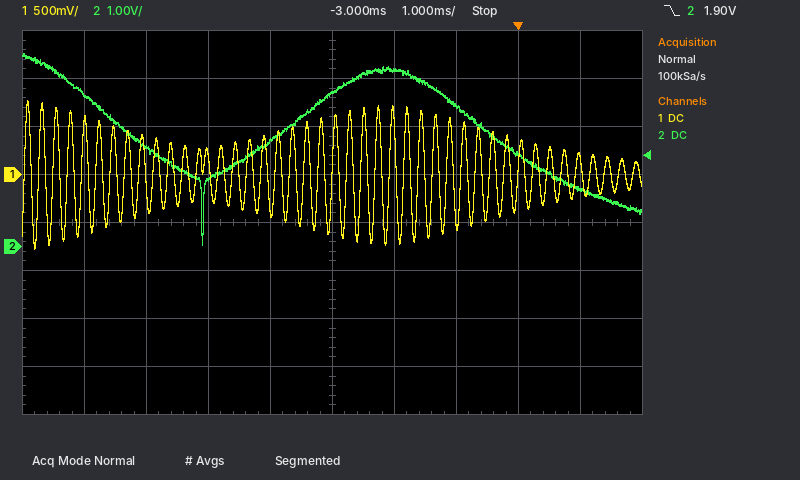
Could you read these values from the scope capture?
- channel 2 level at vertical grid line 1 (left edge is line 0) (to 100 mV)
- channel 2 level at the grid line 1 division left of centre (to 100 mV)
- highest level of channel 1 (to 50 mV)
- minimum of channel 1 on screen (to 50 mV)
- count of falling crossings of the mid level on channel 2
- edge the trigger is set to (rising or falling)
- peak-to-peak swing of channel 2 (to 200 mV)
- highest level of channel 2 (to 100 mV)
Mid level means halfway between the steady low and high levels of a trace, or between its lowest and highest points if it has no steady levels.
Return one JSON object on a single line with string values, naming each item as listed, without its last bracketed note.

{"channel 2 level at vertical grid line 1 (left edge is line 0)": "3.2 V", "channel 2 level at the grid line 1 division left of centre": "2.2 V", "highest level of channel 1": "750 mV", "minimum of channel 1 on screen": "-750 mV", "count of falling crossings of the mid level on channel 2": "2", "edge the trigger is set to": "falling", "peak-to-peak swing of channel 2": "4.0 V", "highest level of channel 2": "4.0 V"}
